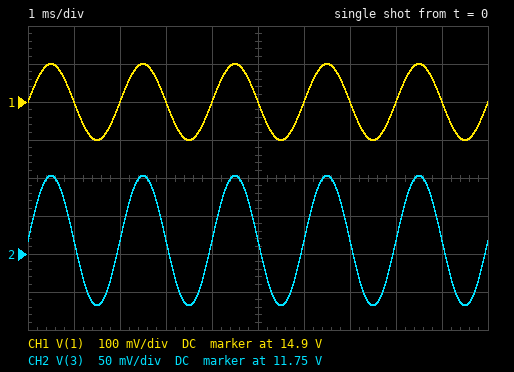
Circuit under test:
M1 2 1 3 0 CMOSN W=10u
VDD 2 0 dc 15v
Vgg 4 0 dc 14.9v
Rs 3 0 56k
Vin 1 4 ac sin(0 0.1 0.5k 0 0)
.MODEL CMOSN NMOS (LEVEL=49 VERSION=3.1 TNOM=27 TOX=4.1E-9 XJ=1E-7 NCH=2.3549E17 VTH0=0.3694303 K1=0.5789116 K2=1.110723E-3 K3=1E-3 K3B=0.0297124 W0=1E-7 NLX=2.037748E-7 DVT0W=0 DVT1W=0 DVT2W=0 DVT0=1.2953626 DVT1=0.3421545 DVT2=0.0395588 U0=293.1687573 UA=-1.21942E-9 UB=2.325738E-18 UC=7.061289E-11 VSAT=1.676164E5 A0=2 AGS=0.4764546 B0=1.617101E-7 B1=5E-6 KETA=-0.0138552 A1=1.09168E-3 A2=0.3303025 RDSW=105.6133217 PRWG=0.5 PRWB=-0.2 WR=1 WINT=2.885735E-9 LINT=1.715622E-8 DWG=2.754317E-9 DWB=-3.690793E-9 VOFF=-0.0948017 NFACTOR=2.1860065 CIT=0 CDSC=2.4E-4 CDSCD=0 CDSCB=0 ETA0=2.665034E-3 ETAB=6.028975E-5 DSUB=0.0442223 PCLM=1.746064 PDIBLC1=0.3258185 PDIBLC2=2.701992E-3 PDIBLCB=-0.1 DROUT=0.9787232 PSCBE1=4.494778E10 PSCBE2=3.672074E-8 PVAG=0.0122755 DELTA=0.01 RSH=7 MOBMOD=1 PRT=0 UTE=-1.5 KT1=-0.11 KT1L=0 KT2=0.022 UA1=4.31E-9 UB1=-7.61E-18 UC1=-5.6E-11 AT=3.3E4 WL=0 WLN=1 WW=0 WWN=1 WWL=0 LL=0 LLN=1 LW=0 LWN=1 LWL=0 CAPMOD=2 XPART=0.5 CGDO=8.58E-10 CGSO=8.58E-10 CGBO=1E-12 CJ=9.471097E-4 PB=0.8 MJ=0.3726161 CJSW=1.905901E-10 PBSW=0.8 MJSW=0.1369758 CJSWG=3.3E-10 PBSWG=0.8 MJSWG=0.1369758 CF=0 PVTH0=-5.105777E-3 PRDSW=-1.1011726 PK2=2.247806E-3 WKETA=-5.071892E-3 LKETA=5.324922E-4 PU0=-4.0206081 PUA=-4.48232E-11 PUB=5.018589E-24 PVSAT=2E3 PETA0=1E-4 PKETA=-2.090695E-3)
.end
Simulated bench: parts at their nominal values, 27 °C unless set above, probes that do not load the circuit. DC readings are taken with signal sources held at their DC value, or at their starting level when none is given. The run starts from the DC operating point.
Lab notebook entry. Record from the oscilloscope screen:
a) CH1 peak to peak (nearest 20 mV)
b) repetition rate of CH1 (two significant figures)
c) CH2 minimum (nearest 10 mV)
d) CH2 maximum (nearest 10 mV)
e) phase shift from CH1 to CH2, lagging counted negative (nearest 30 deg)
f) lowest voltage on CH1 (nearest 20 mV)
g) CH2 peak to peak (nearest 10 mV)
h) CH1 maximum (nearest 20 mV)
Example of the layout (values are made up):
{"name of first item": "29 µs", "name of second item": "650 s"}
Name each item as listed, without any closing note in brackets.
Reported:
{"CH1 peak to peak": "200 mV", "repetition rate of CH1": "500 Hz", "CH2 minimum": "11.68 V", "CH2 maximum": "11.85 V", "phase shift from CH1 to CH2, lagging counted negative": "0 deg", "lowest voltage on CH1": "14.80 V", "CH2 peak to peak": "170 mV", "CH1 maximum": "15.00 V"}
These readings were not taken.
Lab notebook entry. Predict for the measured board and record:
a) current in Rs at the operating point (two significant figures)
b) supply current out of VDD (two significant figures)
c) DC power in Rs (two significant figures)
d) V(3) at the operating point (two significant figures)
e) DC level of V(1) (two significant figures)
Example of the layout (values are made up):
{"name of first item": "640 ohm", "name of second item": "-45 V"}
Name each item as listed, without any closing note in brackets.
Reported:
{"current in Rs at the operating point": "210 µA", "supply current out of VDD": "210 µA", "DC power in Rs": "2.5 mW", "V(3) at the operating point": "12 V", "DC level of V(1)": "15 V"}
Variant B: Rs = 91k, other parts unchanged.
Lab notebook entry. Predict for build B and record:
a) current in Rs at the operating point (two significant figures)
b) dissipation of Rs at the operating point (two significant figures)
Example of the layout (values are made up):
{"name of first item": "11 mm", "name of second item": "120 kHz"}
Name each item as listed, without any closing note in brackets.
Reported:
{"current in Rs at the operating point": "130 µA", "dissipation of Rs at the operating point": "1.6 mW"}
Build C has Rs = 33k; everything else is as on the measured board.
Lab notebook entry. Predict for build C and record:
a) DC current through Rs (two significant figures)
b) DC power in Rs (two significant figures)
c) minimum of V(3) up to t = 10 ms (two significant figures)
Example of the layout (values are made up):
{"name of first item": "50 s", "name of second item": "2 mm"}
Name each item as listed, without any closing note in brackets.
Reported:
{"DC current through Rs": "340 µA", "DC power in Rs": "3.9 mW", "minimum of V(3) up to t = 10 ms": "11 V"}
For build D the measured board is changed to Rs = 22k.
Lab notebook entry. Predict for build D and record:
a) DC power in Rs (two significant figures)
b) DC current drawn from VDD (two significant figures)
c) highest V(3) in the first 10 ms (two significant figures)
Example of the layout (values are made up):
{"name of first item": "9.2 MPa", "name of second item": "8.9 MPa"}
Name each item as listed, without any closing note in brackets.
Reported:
{"DC power in Rs": "5.3 mW", "DC current drawn from VDD": "490 µA", "highest V(3) in the first 10 ms": "11 V"}
